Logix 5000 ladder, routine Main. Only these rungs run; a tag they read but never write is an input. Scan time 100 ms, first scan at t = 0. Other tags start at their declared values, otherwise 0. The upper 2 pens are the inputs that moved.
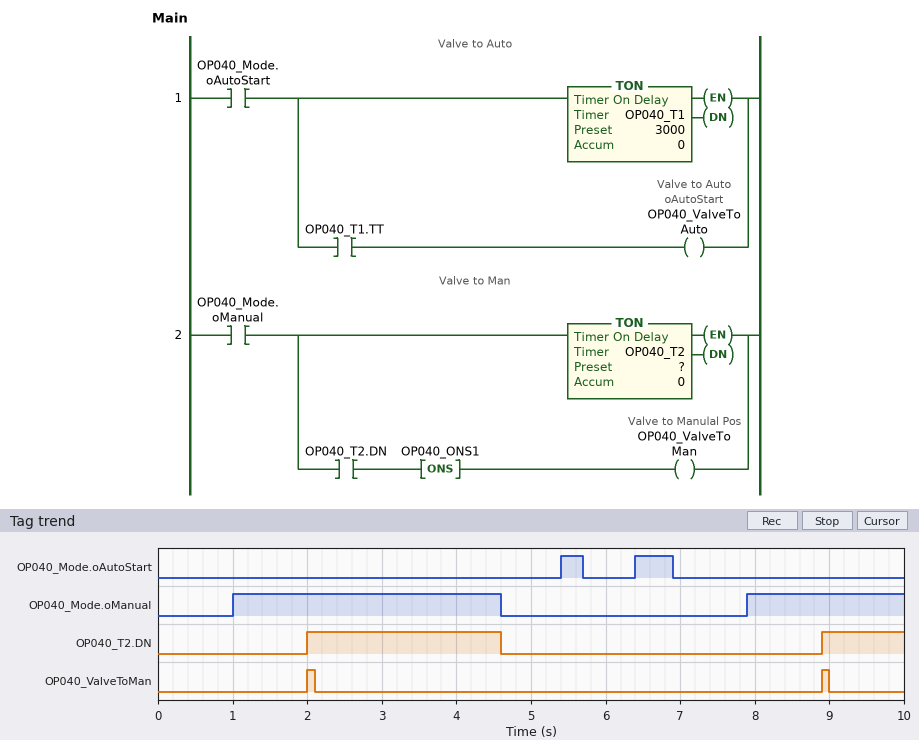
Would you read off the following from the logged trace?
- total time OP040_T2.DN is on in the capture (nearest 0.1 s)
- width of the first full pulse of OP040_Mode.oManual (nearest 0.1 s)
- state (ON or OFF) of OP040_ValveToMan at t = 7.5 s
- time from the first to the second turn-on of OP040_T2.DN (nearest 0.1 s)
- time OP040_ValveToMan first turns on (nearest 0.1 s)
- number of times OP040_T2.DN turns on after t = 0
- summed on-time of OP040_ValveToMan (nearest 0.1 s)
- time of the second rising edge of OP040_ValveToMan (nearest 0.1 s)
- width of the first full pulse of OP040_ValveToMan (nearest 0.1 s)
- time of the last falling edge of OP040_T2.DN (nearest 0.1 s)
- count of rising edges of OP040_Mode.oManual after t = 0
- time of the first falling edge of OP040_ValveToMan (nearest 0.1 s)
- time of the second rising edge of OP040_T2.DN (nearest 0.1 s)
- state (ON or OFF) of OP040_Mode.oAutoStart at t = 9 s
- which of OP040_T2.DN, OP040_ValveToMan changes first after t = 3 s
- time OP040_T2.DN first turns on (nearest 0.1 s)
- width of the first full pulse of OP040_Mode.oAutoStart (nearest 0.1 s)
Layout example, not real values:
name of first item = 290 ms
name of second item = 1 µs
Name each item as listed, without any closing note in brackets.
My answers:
total time OP040_T2.DN is on in the capture = 3.7 s
width of the first full pulse of OP040_Mode.oManual = 3.6 s
state (ON or OFF) of OP040_ValveToMan at t = 7.5 s = OFF
time from the first to the second turn-on of OP040_T2.DN = 6.9 s
time OP040_ValveToMan first turns on = 2.0 s
number of times OP040_T2.DN turns on after t = 0 = 2
summed on-time of OP040_ValveToMan = 0.2 s
time of the second rising edge of OP040_ValveToMan = 8.9 s
width of the first full pulse of OP040_ValveToMan = 0.1 s
time of the last falling edge of OP040_T2.DN = 4.6 s
count of rising edges of OP040_Mode.oManual after t = 0 = 2
time of the first falling edge of OP040_ValveToMan = 2.1 s
time of the second rising edge of OP040_T2.DN = 8.9 s
state (ON or OFF) of OP040_Mode.oAutoStart at t = 9 s = OFF
which of OP040_T2.DN, OP040_ValveToMan changes first after t = 3 s = OP040_T2.DN
time OP040_T2.DN first turns on = 2.0 s
width of the first full pulse of OP040_Mode.oAutoStart = 0.3 s
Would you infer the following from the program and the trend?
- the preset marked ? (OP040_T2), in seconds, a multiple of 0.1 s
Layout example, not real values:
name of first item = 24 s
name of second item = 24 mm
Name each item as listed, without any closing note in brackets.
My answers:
the preset marked ? (OP040_T2), in seconds, a multiple of 0.1 s = 1.0 s
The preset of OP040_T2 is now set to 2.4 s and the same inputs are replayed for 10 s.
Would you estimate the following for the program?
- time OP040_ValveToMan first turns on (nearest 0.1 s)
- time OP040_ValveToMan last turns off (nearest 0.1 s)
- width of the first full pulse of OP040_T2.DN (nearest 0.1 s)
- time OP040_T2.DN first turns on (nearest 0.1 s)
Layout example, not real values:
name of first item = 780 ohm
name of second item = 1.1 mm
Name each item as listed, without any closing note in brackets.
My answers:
time OP040_ValveToMan first turns on = 3.4 s
time OP040_ValveToMan last turns off = 3.5 s
width of the first full pulse of OP040_T2.DN = 1.2 s
time OP040_T2.DN first turns on = 3.4 s
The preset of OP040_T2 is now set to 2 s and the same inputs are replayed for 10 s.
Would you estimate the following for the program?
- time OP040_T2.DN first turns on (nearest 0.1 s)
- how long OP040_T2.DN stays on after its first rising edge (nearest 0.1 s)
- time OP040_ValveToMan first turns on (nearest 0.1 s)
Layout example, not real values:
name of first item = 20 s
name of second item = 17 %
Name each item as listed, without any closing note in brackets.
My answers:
time OP040_T2.DN first turns on = 3.0 s
how long OP040_T2.DN stays on after its first rising edge = 1.6 s
time OP040_ValveToMan first turns on = 3.0 s
